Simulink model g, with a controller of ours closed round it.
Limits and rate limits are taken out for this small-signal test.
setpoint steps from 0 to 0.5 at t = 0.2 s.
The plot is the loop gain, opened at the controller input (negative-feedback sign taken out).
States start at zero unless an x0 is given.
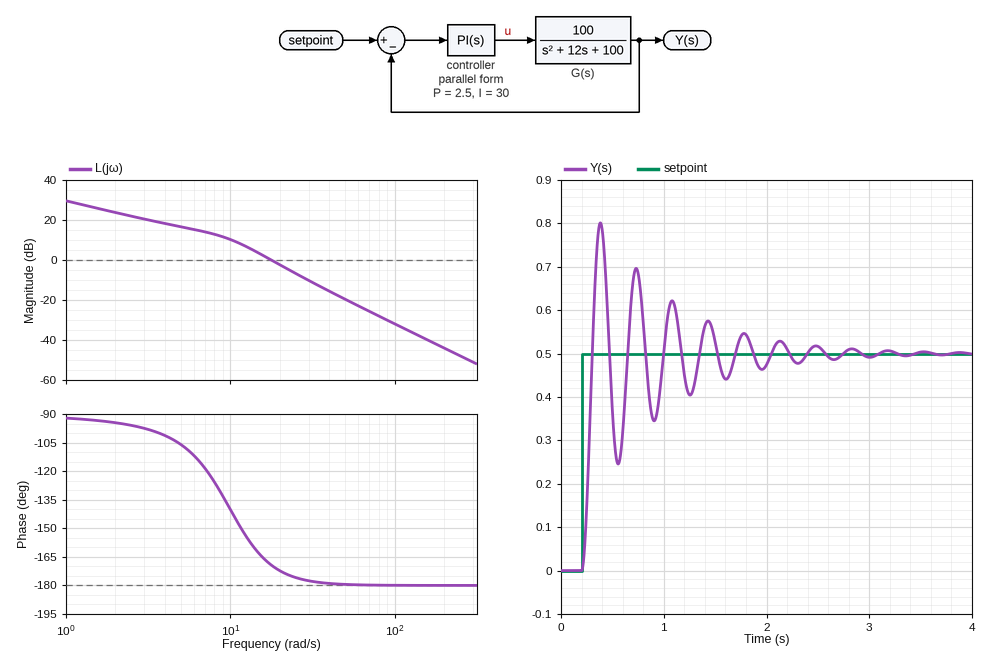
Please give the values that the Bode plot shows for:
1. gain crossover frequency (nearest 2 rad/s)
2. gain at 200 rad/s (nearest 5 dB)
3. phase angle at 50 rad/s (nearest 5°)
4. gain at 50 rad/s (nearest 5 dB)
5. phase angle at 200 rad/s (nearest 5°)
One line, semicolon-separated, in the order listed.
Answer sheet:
18 rad/s; -45 dB; -180°; -20 dB; -180°
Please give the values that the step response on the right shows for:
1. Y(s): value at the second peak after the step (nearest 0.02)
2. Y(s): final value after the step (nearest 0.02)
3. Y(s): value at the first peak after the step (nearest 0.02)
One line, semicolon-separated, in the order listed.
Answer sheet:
0.70; 0.50; 0.80
